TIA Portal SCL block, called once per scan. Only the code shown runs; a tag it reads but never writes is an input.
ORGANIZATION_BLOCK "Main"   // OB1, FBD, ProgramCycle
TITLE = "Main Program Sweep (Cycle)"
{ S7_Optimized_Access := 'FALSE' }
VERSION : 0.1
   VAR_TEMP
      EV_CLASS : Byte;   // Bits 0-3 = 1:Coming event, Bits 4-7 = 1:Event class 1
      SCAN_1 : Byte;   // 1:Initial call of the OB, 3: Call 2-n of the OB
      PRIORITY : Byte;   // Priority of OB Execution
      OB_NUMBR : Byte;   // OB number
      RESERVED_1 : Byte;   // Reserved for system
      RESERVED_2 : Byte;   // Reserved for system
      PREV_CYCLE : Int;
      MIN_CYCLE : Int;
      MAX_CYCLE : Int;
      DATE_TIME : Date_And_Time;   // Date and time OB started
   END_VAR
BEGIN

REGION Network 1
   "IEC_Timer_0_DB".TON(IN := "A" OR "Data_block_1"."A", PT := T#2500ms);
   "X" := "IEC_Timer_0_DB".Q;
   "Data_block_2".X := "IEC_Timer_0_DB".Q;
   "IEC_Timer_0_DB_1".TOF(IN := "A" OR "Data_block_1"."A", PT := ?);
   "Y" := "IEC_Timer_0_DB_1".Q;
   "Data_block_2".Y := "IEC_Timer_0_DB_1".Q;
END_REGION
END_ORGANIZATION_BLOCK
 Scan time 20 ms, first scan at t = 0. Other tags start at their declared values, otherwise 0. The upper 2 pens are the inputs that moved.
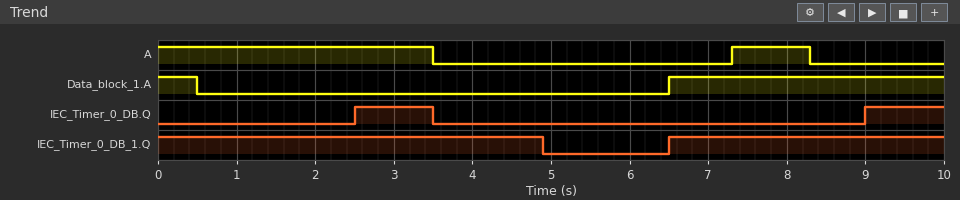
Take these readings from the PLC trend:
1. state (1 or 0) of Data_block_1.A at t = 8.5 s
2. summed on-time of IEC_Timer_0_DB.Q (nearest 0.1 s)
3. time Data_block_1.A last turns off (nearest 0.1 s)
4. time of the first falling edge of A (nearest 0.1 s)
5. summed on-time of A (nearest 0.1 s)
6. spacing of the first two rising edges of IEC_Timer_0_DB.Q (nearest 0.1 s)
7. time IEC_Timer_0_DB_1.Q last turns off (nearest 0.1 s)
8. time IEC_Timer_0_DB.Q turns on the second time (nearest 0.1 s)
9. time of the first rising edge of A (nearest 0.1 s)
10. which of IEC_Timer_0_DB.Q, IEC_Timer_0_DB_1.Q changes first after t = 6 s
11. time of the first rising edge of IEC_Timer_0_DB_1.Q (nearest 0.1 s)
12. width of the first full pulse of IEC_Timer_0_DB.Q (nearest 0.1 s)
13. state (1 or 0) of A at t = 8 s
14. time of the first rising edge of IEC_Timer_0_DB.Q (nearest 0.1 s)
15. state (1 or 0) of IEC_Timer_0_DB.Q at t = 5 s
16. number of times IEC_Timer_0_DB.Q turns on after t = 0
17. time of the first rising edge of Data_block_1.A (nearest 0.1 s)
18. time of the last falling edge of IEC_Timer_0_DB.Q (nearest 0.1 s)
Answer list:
1
2.0 s
0.5 s
3.5 s
4.5 s
6.5 s
4.9 s
9.0 s
7.3 s
IEC_Timer_0_DB_1.Q
6.5 s
1.0 s
1
2.5 s
0
2
6.5 s
3.5 s
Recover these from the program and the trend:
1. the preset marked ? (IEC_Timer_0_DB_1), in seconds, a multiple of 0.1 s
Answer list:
1.4 s
